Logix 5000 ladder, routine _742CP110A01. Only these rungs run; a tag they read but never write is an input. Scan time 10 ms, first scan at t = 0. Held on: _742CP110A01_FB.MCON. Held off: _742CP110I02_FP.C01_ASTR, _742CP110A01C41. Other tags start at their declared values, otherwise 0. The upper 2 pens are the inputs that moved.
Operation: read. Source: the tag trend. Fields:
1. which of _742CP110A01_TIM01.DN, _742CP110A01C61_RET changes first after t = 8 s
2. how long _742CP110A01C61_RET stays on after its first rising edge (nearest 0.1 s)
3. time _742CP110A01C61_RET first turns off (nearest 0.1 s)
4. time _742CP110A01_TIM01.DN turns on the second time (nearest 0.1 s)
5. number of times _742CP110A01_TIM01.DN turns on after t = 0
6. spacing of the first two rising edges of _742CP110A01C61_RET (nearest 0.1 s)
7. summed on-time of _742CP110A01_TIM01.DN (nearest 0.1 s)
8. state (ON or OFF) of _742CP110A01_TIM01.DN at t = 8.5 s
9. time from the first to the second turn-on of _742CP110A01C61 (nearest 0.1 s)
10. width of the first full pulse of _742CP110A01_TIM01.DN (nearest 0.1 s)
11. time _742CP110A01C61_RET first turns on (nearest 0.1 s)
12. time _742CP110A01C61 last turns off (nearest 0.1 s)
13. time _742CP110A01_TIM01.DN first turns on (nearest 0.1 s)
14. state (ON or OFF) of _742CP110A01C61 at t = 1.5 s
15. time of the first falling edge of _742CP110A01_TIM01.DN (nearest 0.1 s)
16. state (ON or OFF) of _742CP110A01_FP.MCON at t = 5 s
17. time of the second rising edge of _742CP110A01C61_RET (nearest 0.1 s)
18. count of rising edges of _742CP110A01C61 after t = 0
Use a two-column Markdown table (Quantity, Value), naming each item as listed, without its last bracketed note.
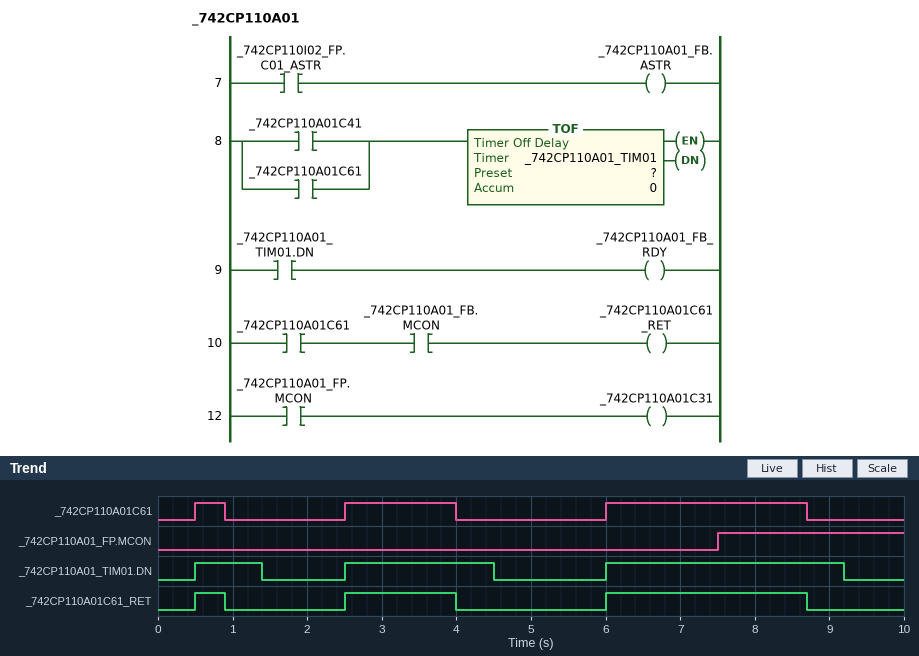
| Quantity | Value |
|---|---|
| which of _742CP110A01_TIM01.DN, _742CP110A01C61_RET changes first after t = 8 s | _742CP110A01C61_RET |
| how long _742CP110A01C61_RET stays on after its first rising edge | 0.4 s |
| time _742CP110A01C61_RET first turns off | 0.9 s |
| time _742CP110A01_TIM01.DN turns on the second time | 2.5 s |
| number of times _742CP110A01_TIM01.DN turns on after t = 0 | 3 |
| spacing of the first two rising edges of _742CP110A01C61_RET | 2.0 s |
| summed on-time of _742CP110A01_TIM01.DN | 6.1 s |
| state (ON or OFF) of _742CP110A01_TIM01.DN at t = 8.5 s | ON |
| time from the first to the second turn-on of _742CP110A01C61 | 2.0 s |
| width of the first full pulse of _742CP110A01_TIM01.DN | 0.9 s |
| time _742CP110A01C61_RET first turns on | 0.5 s |
| time _742CP110A01C61 last turns off | 8.7 s |
| time _742CP110A01_TIM01.DN first turns on | 0.5 s |
| state (ON or OFF) of _742CP110A01C61 at t = 1.5 s | OFF |
| time of the first falling edge of _742CP110A01_TIM01.DN | 1.4 s |
| state (ON or OFF) of _742CP110A01_FP.MCON at t = 5 s | OFF |
| time of the second rising edge of _742CP110A01C61_RET | 2.5 s |
| count of rising edges of _742CP110A01C61 after t = 0 | 3 |
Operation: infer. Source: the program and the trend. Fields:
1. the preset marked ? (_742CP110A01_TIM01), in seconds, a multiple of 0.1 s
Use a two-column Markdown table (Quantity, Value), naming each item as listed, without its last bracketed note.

| Quantity | Value |
|---|---|
| the preset marked ? (_742CP110A01_TIM01), in seconds, a multiple of 0.1 s | 0.5 s |
